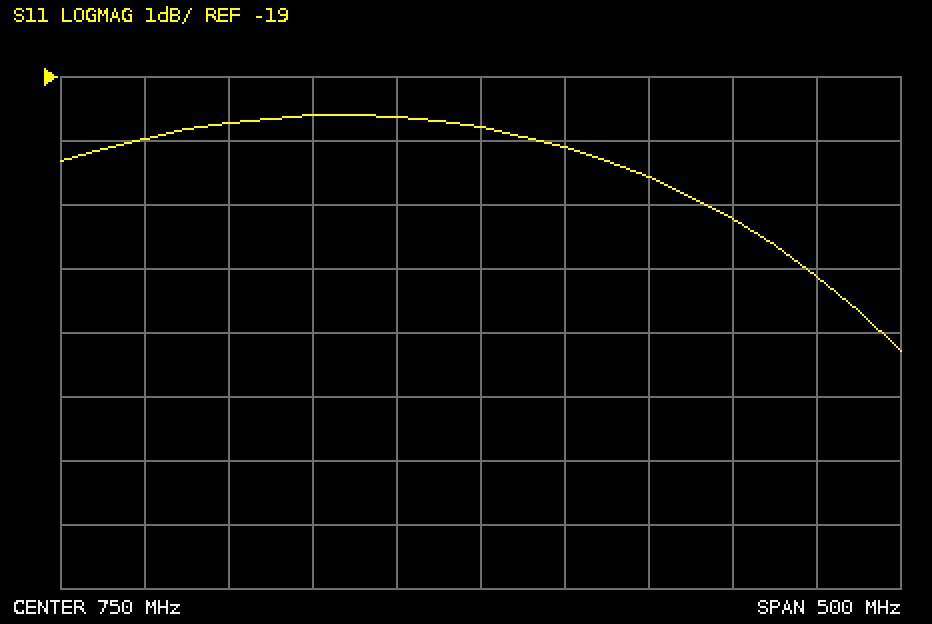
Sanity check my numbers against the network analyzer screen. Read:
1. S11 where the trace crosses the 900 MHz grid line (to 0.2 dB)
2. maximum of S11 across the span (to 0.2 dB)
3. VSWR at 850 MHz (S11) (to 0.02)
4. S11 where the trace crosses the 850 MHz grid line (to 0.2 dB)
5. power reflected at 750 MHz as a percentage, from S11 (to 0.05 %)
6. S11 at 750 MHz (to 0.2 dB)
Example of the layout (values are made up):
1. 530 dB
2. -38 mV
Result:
1. -21.2 dB
2. -19.6 dB
3. 1.20
4. -20.6 dB
5. 1.05 %
6. -19.8 dB
